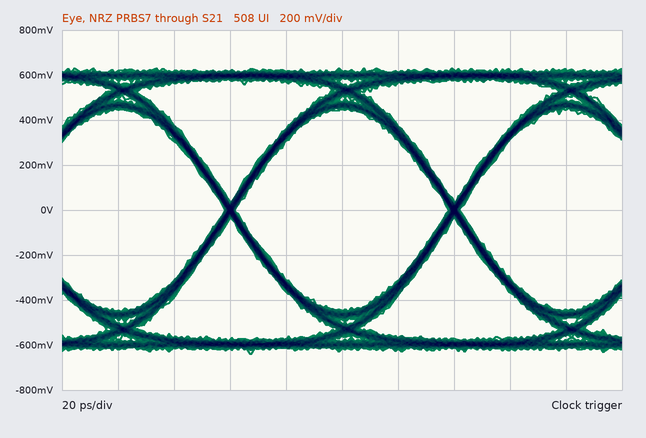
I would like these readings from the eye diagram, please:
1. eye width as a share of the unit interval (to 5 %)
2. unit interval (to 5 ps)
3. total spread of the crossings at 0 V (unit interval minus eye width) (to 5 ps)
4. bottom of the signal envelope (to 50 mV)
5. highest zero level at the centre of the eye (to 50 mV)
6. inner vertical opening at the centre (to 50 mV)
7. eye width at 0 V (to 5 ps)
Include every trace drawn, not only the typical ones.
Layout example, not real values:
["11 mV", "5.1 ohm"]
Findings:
["95 %", "80 ps", "5 ps", "-650 mV", "-450 mV", "900 mV", "75 ps"]
